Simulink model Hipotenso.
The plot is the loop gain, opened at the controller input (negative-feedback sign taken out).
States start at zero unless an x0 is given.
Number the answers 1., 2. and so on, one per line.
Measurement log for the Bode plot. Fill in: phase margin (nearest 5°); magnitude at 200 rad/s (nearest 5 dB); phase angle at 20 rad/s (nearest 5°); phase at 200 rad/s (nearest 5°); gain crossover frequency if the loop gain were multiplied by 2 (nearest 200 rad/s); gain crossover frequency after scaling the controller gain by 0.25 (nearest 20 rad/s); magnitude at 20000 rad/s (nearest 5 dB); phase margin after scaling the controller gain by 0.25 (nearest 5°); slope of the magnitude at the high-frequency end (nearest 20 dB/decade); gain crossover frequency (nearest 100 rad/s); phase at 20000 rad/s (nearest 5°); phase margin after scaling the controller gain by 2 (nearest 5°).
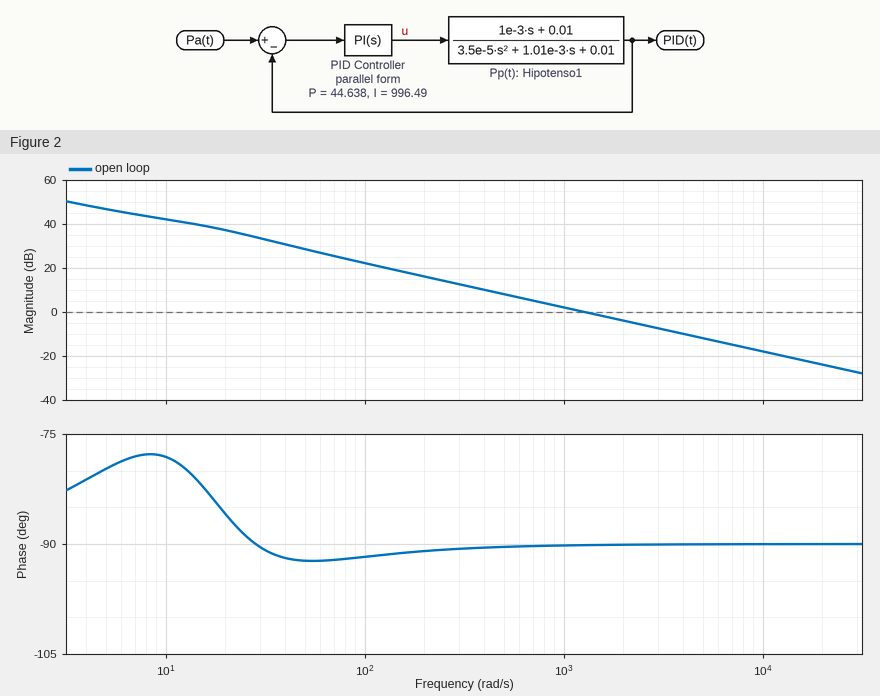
1. 90°
2. 15 dB
3. -85°
4. -90°
5. 2600 rad/s
6. 320 rad/s
7. -25 dB
8. 90°
9. -20 dB/decade
10. 1300 rad/s
11. -90°
12. 90°
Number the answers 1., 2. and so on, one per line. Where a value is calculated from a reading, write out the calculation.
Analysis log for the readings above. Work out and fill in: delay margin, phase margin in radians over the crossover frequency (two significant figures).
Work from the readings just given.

1. 90 × π / 180 / 1300 = 0.0012 s
